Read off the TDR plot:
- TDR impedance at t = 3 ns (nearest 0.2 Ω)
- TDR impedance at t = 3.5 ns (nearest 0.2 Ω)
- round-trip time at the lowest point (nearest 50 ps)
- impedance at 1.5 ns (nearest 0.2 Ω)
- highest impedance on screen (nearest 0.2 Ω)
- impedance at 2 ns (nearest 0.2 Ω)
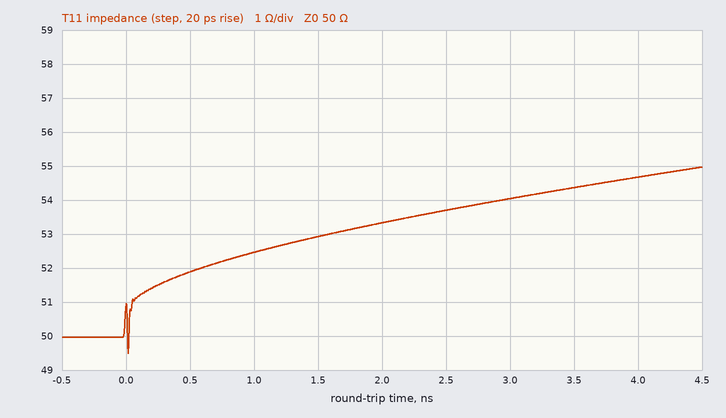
54.0 Ω
54.4 Ω
0 ps
53.0 Ω
55.0 Ω
53.4 Ω
